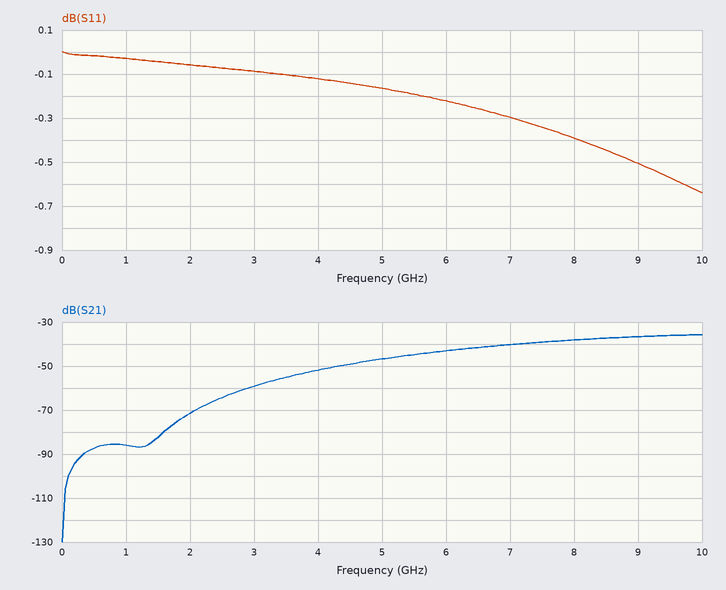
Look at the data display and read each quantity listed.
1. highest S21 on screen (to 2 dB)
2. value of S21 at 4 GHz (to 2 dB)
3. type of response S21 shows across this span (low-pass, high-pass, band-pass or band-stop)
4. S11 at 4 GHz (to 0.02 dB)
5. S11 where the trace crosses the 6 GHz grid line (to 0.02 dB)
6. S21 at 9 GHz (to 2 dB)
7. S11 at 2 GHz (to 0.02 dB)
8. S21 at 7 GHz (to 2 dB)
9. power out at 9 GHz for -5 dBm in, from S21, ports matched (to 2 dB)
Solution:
-36 dB
-52 dB
high-pass
-0.12 dB
-0.22 dB
-36 dB
-0.06 dB
-40 dB
-42 dBm
